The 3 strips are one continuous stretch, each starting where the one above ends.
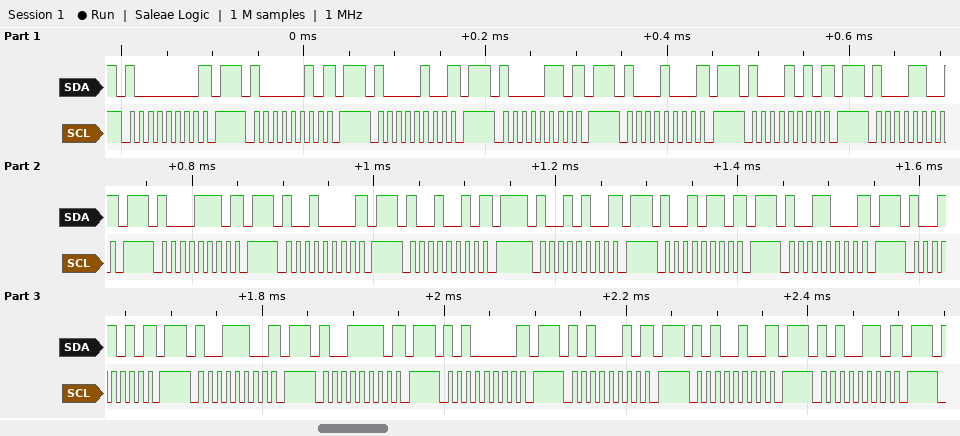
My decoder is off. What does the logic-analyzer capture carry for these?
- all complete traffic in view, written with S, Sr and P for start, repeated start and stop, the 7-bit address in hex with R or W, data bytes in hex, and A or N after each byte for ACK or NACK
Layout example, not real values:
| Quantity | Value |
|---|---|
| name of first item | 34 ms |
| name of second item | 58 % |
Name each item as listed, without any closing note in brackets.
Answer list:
| Quantity | Value |
|---|---|
| all complete traffic in view, written with S, Sr and P for start, repeated start and stop, the 7-bit address in hex with R or W, data bytes in hex, and A or N after each byte for ACK or NACK | S 40W N P S 41W N P S 42W N P S 43W N P S 44W N P S 45W N P S 46W N P S 47W N P S 48W N P S 49W N P S 4AW N P S 4BW N P S 4CW N P S 4DW N P S 4EW N P S 4FW N P S 50W N P S 51W N P S 52W N P S 53W N P |
